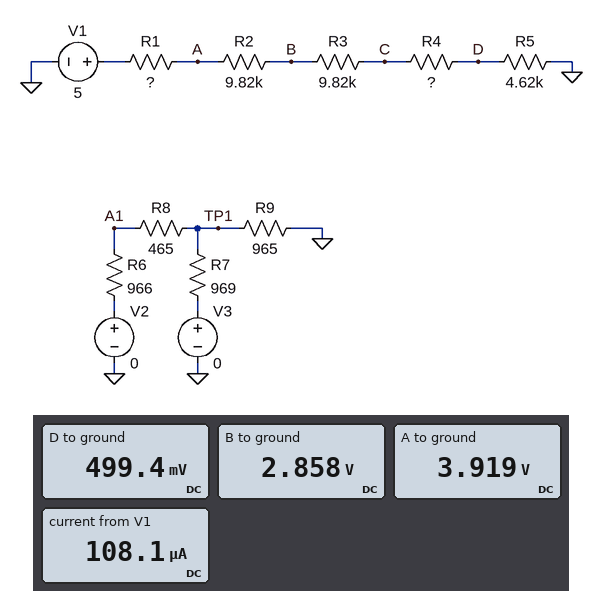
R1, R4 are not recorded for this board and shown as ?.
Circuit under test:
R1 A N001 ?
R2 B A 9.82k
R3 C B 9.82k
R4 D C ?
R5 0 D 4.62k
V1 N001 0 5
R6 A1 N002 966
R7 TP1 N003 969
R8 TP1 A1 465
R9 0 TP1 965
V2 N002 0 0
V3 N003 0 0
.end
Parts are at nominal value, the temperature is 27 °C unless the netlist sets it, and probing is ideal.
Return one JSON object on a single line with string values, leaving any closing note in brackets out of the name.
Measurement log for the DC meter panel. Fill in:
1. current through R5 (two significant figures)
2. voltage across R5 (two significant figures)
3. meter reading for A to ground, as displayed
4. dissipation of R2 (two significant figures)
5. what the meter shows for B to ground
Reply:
{"current through R5": "110 µA", "voltage across R5": "500 mV", "meter reading for A to ground, as displayed": "3.919 V", "dissipation of R2": "110 µW", "what the meter shows for B to ground": "2.858 V"}
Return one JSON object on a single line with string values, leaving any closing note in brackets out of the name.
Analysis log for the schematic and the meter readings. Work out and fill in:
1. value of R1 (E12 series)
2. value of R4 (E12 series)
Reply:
{"value of R1": "10 kΩ", "value of R4": "12 kΩ"}
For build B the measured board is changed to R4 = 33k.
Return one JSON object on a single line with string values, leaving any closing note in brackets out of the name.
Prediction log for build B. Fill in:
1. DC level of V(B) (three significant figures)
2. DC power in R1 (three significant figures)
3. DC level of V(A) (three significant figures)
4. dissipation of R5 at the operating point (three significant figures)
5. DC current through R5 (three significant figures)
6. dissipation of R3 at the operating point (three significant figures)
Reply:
{"DC level of V(B)": "3.53 V", "DC power in R1": "55.3 µW", "DC level of V(A)": "4.26 V", "dissipation of R5 at the operating point": "25.5 µW", "DC current through R5": "74.3 µA", "dissipation of R3 at the operating point": "54.3 µW"}
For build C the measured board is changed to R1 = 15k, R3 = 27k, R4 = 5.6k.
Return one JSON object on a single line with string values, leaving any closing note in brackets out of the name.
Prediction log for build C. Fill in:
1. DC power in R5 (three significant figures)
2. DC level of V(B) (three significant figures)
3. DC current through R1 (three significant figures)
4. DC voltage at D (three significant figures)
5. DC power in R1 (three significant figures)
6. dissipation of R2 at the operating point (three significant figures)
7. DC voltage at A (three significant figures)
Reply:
{"DC power in R5": "30.0 µW", "DC level of V(B)": "3.00 V", "DC current through R1": "80.6 µA", "DC voltage at D": "372 mV", "DC power in R1": "97.4 µW", "dissipation of R2 at the operating point": "63.8 µW", "DC voltage at A": "3.79 V"}
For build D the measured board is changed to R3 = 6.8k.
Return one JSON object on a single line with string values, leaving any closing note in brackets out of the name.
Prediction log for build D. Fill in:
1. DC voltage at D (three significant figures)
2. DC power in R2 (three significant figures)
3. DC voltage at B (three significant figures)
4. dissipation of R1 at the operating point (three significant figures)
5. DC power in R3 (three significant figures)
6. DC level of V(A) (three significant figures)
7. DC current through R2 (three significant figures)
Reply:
{"DC voltage at D": "534 mV", "DC power in R2": "131 µW", "DC voltage at B": "2.71 V", "dissipation of R1 at the operating point": "134 µW", "DC power in R3": "90.9 µW", "DC level of V(A)": "3.84 V", "DC current through R2": "116 µA"}
